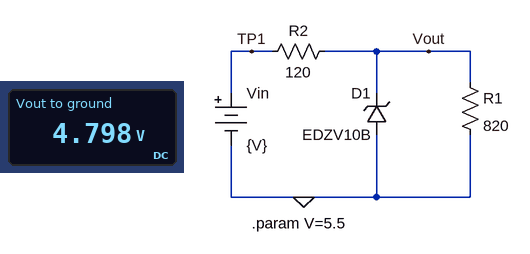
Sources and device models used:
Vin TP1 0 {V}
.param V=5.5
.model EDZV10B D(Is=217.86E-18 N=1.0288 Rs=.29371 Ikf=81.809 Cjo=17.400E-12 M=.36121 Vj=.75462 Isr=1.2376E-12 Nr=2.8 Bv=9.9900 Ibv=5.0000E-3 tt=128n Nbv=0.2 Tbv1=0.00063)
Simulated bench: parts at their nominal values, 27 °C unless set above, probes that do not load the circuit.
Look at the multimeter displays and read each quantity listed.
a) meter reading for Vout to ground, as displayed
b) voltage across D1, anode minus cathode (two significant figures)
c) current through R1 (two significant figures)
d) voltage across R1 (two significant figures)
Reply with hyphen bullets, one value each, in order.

- 4.798 V
- -4.8 V
- 5.9 mA
- 4.8 V
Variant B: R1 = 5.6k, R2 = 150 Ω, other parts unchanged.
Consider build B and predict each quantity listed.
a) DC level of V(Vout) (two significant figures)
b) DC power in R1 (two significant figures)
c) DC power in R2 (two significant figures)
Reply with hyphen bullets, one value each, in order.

- 5.4 V
- 5.1 mW
- 140 µW
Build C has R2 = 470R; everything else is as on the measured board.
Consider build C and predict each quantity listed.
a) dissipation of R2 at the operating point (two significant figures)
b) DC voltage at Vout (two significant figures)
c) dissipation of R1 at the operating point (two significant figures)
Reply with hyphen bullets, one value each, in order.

- 8.5 mW
- 3.5 V
- 15 mW
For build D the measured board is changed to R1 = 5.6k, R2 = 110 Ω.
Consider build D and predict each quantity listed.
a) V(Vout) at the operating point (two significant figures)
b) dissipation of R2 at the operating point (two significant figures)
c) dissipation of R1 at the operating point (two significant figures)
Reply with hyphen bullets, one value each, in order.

- 5.4 V
- 100 µW
- 5.2 mW
